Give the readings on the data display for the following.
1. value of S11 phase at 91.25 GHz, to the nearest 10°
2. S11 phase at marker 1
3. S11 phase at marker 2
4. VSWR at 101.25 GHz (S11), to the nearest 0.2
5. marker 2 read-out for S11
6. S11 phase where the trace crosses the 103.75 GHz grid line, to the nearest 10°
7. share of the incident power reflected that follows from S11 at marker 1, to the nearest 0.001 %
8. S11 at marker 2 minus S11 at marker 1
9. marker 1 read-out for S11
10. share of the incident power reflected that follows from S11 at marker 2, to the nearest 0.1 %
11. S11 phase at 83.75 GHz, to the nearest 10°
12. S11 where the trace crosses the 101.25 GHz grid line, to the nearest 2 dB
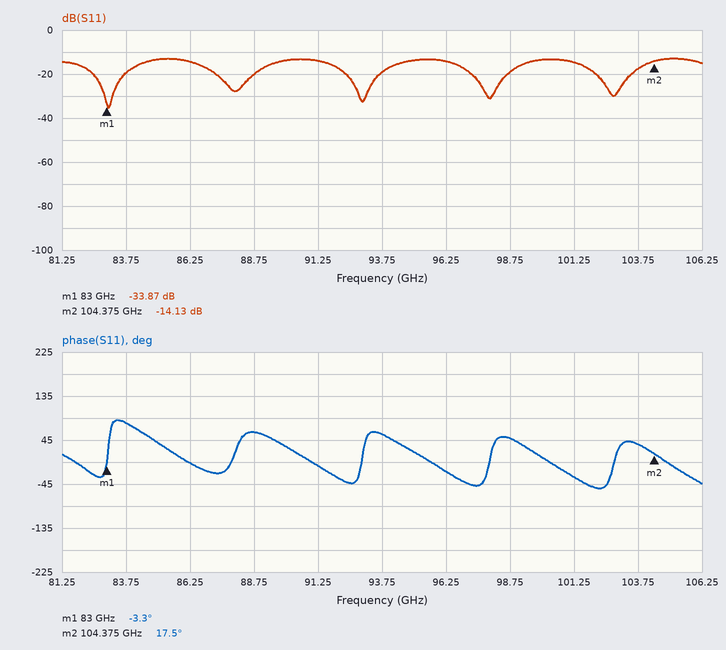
-10°
-3.3°
17.5°
1.4
-14.13 dB
40°
0.041 %
19.74 dB
-33.87 dB
3.9 %
80°
-14 dB
